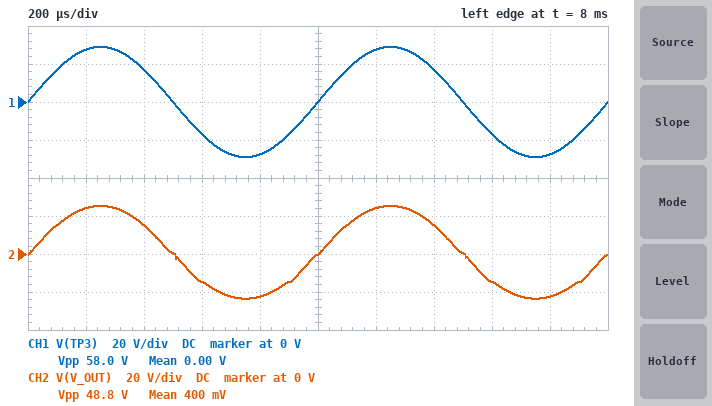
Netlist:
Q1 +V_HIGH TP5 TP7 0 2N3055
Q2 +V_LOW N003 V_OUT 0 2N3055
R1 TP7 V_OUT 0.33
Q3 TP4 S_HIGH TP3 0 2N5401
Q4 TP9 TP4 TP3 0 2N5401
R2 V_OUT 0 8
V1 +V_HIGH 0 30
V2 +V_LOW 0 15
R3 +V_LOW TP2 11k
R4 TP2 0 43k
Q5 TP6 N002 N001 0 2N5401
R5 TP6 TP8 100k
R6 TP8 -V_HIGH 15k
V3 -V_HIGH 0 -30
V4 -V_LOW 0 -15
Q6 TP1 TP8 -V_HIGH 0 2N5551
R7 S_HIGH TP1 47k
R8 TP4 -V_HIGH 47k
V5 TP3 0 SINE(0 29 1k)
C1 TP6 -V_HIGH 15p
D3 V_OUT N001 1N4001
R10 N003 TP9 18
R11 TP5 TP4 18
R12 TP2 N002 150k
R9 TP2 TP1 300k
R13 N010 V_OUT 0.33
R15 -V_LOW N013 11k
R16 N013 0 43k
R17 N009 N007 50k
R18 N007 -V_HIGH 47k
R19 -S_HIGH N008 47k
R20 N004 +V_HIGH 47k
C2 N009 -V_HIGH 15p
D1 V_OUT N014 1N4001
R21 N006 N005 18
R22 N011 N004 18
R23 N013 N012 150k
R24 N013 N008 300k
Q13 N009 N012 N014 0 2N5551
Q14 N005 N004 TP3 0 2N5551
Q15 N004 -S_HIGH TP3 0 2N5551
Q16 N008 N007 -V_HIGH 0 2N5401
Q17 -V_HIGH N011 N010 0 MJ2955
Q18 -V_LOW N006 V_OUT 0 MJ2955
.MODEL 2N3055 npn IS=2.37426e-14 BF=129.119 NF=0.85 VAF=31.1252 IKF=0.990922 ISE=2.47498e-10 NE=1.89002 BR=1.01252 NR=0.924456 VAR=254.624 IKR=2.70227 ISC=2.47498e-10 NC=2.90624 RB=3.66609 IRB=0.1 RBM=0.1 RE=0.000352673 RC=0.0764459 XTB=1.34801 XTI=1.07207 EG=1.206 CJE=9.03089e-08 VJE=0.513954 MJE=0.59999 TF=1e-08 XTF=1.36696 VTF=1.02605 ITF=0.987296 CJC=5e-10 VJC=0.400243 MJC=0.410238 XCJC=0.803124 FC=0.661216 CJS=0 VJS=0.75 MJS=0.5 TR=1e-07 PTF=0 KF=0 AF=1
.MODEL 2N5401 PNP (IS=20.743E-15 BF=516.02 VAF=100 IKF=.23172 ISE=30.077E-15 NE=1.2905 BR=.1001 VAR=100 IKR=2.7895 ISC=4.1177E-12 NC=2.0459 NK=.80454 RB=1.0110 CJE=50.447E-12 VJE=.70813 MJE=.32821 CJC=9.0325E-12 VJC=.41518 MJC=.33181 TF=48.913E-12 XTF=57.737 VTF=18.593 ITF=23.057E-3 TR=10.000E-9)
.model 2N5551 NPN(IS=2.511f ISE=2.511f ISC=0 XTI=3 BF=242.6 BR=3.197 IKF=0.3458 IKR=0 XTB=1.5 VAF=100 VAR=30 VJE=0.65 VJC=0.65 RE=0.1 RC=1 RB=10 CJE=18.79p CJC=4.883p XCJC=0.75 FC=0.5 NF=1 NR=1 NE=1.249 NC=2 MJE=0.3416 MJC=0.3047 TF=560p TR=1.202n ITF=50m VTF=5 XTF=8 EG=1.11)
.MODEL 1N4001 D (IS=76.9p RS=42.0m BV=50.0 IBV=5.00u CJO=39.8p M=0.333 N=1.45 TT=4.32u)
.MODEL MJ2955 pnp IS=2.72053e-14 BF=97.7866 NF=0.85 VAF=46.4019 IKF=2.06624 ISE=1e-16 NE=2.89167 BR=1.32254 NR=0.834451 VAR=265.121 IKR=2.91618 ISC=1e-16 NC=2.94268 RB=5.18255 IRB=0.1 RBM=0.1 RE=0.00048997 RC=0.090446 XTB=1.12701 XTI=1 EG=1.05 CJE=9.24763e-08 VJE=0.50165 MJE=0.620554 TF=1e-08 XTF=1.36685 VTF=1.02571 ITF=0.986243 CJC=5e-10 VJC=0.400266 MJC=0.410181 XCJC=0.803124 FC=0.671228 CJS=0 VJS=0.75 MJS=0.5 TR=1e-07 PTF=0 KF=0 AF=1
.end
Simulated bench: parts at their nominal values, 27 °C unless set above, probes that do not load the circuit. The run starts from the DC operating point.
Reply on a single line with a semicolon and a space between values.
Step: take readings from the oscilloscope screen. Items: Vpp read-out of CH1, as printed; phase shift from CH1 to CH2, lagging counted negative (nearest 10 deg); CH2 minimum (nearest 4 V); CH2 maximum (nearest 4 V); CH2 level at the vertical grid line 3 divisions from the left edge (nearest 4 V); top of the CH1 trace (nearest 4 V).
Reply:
58.0 V; 0 deg; -24 V; 24 V; -16 V; 28 V
